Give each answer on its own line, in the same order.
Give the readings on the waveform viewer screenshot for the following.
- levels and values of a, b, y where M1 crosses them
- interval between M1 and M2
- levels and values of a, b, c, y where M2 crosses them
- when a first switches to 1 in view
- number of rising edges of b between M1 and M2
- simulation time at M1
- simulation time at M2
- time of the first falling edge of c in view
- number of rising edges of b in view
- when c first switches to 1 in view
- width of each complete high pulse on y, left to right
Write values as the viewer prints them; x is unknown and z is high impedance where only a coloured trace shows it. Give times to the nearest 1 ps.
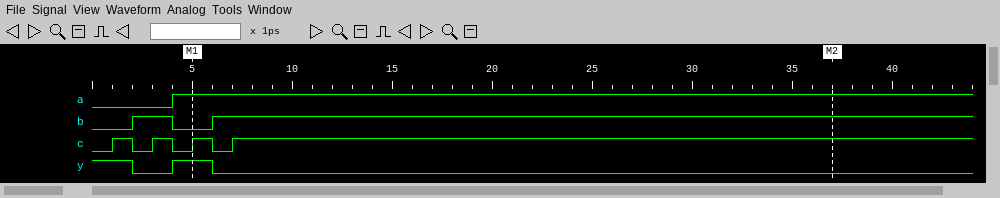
a=1, b=0, y=1
32 ps
a=1, b=1, c=1, y=0
4 ps
1
5 ps
37 ps
2 ps
2
1 ps
2 ps
